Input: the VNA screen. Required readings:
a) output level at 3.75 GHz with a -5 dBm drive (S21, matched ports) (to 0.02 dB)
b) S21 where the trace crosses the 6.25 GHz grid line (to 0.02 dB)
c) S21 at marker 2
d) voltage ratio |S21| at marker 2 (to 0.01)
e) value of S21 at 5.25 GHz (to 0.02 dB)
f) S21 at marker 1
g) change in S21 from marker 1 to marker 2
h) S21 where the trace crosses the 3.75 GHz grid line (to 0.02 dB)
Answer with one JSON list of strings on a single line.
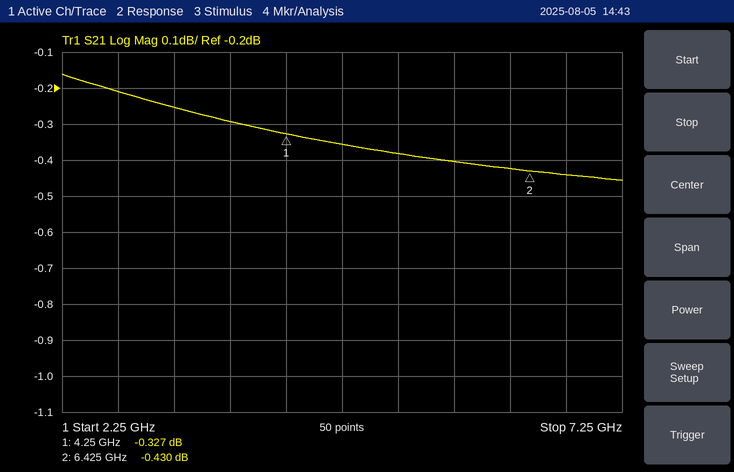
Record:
["-5.30 dBm", "-0.42 dB", "-0.430 dB", "0.95", "-0.38 dB", "-0.327 dB", "-0.103 dB", "-0.30 dB"]
